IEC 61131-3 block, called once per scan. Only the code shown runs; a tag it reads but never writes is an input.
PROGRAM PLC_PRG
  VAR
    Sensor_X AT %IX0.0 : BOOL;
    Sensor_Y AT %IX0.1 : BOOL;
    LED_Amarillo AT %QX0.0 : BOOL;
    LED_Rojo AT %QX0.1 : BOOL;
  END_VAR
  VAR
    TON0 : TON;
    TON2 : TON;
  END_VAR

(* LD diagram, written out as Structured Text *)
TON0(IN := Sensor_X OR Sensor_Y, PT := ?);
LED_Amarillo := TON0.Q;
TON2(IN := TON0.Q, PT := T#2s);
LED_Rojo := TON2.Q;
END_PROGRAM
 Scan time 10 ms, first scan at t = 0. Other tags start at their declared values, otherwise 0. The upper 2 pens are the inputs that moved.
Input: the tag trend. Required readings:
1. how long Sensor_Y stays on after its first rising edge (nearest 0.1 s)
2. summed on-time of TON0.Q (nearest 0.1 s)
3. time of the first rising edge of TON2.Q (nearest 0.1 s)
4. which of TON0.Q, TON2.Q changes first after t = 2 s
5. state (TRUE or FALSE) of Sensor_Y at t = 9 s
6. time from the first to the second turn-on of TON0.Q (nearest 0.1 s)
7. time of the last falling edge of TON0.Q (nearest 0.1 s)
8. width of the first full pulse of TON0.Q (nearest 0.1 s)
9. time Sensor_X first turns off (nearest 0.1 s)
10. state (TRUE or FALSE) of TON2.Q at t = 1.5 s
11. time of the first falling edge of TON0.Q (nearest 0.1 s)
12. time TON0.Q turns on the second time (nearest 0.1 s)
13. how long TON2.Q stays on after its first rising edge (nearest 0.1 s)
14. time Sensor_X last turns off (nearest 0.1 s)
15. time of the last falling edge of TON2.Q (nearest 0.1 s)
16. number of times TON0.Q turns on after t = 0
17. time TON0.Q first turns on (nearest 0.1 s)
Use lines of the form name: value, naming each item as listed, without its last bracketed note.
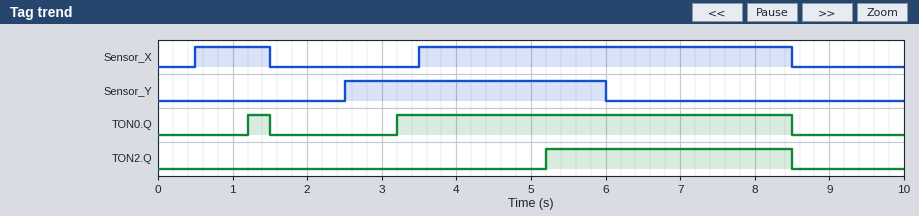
how long Sensor_Y stays on after its first rising edge: 3.5 s
summed on-time of TON0.Q: 5.6 s
time of the first rising edge of TON2.Q: 5.2 s
which of TON0.Q, TON2.Q changes first after t = 2 s: TON0.Q
state (TRUE or FALSE) of Sensor_Y at t = 9 s: FALSE
time from the first to the second turn-on of TON0.Q: 2.0 s
time of the last falling edge of TON0.Q: 8.5 s
width of the first full pulse of TON0.Q: 0.3 s
time Sensor_X first turns off: 1.5 s
state (TRUE or FALSE) of TON2.Q at t = 1.5 s: FALSE
time of the first falling edge of TON0.Q: 1.5 s
time TON0.Q turns on the second time: 3.2 s
how long TON2.Q stays on after its first rising edge: 3.3 s
time Sensor_X last turns off: 8.5 s
time of the last falling edge of TON2.Q: 8.5 s
number of times TON0.Q turns on after t = 0: 2
time TON0.Q first turns on: 1.2 s
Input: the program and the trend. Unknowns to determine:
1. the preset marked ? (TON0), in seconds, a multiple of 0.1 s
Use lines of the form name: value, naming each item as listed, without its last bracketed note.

the preset marked ? (TON0), in seconds, a multiple of 0.1 s: 0.7 s
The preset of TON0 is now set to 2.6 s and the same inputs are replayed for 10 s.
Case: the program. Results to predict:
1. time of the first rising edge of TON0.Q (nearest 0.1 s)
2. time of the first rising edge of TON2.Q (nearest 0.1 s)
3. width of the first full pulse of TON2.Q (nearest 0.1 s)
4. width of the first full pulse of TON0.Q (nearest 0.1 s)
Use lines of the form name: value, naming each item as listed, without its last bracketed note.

time of the first rising edge of TON0.Q: 5.1 s
time of the first rising edge of TON2.Q: 7.1 s
width of the first full pulse of TON2.Q: 1.4 s
width of the first full pulse of TON0.Q: 3.4 s
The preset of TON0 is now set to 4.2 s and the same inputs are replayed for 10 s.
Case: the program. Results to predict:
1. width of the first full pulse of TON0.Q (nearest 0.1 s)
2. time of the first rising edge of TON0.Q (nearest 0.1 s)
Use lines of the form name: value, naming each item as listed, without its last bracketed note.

width of the first full pulse of TON0.Q: 1.8 s
time of the first rising edge of TON0.Q: 6.7 s
